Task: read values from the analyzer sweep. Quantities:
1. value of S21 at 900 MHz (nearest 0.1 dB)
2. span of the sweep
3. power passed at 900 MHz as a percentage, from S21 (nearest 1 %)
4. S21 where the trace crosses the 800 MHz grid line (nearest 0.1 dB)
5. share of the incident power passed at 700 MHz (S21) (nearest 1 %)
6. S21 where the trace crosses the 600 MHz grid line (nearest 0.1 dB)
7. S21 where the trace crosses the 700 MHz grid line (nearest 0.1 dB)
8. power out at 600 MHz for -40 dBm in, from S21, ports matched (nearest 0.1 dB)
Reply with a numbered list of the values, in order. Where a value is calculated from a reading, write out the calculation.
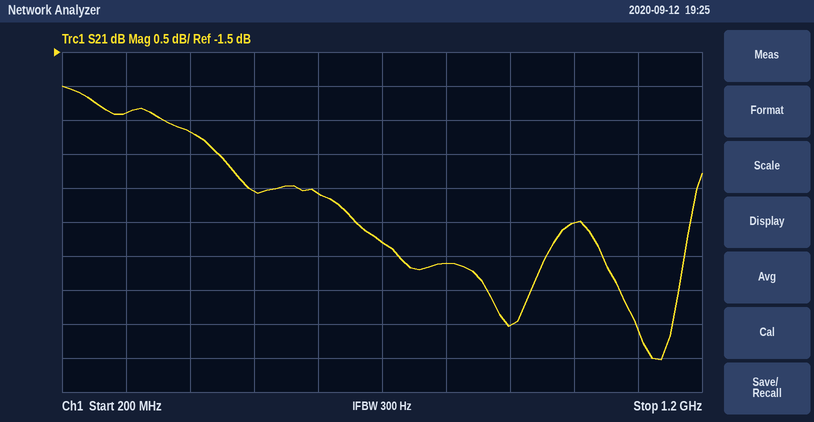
1. -5.5 dB
2. 1 GHz
3. 10^(-5.5/10) ≈ 28 %
4. -4.6 dB
5. 10^(-4.3/10) ≈ 37 %
6. -3.6 dB
7. -4.3 dB
8. -40 dBm + (-3.6 dB) = -43.6 dBm
